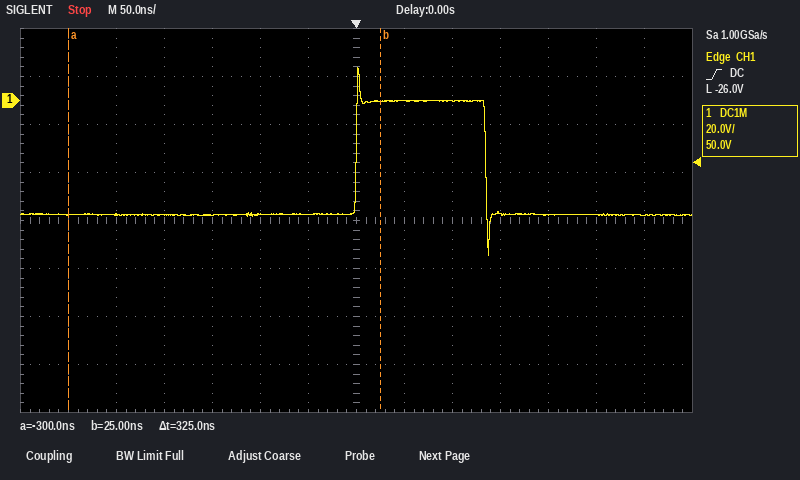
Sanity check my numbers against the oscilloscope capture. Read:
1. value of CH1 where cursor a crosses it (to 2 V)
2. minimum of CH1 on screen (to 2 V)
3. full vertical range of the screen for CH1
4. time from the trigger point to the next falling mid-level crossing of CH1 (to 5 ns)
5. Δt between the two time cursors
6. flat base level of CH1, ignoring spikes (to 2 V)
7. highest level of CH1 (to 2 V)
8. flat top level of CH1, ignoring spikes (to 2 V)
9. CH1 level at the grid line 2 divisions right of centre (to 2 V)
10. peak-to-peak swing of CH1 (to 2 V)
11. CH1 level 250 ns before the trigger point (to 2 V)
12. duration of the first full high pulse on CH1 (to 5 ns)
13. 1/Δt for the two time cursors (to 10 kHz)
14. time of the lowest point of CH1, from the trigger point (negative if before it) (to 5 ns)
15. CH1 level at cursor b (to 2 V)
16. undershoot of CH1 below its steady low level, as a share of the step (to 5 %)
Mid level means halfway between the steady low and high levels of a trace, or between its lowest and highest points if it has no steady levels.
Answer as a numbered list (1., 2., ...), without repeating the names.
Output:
1. -48 V
2. -64 V
3. 160 V
4. 135 ns
5. 325 ns
6. -48 V
7. 14 V
8. 0 V
9. 0 V
10. 78 V
11. -48 V
12. 135 ns
13. 3.08 MHz
14. +140 ns
15. 0 V
16. 35 %
